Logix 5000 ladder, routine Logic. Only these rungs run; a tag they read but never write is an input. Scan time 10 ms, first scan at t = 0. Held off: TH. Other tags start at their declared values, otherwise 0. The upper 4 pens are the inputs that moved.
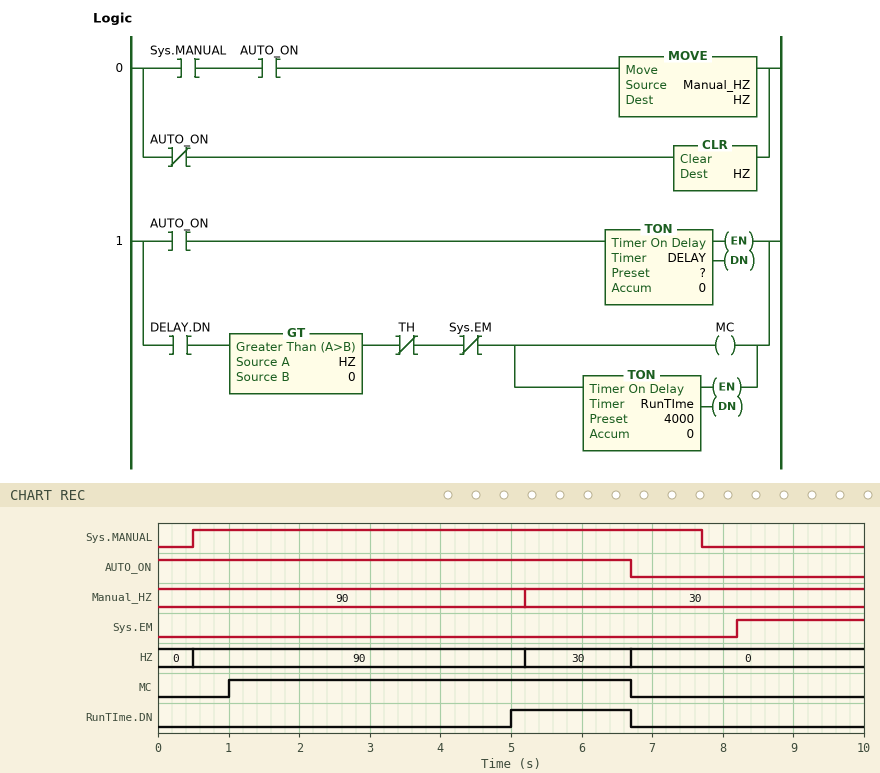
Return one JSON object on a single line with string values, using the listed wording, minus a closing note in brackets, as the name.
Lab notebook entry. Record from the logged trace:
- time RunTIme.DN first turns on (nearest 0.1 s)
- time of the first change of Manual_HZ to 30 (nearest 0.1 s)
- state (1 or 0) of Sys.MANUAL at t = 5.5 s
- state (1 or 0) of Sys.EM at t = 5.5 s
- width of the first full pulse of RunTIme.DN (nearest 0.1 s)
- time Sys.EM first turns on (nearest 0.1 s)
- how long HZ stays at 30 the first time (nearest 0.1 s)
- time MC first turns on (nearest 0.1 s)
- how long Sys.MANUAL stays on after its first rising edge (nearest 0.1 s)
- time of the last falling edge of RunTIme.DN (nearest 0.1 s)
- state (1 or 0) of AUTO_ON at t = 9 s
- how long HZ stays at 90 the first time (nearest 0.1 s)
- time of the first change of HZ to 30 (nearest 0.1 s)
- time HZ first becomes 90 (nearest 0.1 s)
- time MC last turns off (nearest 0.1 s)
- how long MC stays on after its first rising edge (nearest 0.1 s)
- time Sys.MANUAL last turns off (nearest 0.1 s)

{"time RunTIme.DN first turns on": "5.0 s", "time of the first change of Manual_HZ to 30": "5.2 s", "state (1 or 0) of Sys.MANUAL at t = 5.5 s": "1", "state (1 or 0) of Sys.EM at t = 5.5 s": "0", "width of the first full pulse of RunTIme.DN": "1.7 s", "time Sys.EM first turns on": "8.2 s", "how long HZ stays at 30 the first time": "1.5 s", "time MC first turns on": "1.0 s", "how long Sys.MANUAL stays on after its first rising edge": "7.2 s", "time of the last falling edge of RunTIme.DN": "6.7 s", "state (1 or 0) of AUTO_ON at t = 9 s": "0", "how long HZ stays at 90 the first time": "4.7 s", "time of the first change of HZ to 30": "5.2 s", "time HZ first becomes 90": "0.5 s", "time MC last turns off": "6.7 s", "how long MC stays on after its first rising edge": "5.7 s", "time Sys.MANUAL last turns off": "7.7 s"}
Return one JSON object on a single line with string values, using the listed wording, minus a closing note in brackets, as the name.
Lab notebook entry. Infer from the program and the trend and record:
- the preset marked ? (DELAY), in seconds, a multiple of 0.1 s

{"the preset marked ? (DELAY), in seconds, a multiple of 0.1 s": "1.0 s"}
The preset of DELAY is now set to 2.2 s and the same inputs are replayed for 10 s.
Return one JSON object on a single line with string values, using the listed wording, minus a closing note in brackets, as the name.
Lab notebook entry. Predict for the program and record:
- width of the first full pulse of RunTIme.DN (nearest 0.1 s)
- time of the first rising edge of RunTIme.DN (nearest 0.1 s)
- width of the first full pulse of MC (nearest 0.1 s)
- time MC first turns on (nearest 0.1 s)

{"width of the first full pulse of RunTIme.DN": "0.5 s", "time of the first rising edge of RunTIme.DN": "6.2 s", "width of the first full pulse of MC": "4.5 s", "time MC first turns on": "2.2 s"}
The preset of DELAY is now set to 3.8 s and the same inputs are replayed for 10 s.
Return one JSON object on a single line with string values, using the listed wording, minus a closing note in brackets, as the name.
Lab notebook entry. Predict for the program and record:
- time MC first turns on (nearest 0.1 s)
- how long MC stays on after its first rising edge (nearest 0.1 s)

{"time MC first turns on": "3.8 s", "how long MC stays on after its first rising edge": "2.9 s"}
